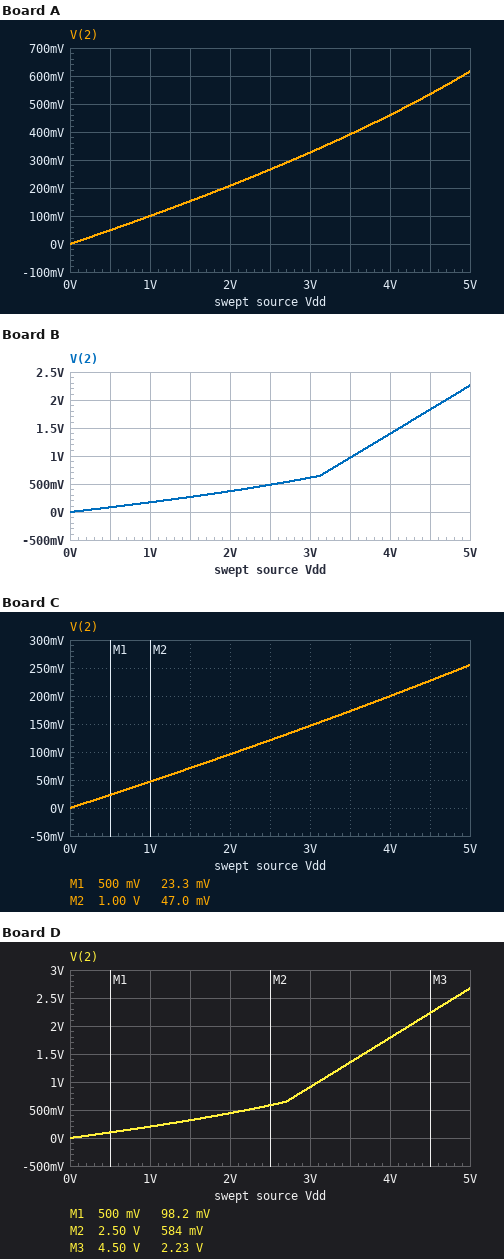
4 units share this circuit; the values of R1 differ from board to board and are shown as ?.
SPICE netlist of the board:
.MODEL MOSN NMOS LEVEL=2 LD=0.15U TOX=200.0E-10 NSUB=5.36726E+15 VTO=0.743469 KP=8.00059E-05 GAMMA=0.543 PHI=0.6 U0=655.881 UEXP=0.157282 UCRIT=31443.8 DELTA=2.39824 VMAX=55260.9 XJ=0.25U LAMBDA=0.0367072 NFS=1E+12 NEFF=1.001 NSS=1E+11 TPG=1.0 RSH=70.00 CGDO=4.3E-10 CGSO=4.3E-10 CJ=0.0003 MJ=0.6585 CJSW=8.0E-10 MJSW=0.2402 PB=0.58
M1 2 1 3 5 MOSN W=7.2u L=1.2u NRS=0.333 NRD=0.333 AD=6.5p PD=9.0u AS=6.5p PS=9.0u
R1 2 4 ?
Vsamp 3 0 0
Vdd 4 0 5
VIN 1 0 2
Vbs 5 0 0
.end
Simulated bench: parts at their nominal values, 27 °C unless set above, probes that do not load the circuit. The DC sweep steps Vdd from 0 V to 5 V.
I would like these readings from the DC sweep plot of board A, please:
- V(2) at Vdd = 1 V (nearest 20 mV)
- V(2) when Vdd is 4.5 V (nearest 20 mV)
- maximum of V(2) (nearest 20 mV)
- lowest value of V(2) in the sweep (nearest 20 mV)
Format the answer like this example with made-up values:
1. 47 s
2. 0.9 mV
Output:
1. 100 mV
2. 540 mV
3. 620 mV
4. 0 V
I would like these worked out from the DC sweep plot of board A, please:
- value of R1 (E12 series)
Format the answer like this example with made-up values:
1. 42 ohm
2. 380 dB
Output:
1. 15 kΩ
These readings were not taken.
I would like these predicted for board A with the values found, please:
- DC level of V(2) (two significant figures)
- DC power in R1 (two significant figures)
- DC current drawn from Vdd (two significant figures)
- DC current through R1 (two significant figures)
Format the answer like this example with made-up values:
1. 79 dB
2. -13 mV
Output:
1. 620 mV
2. 1.3 mW
3. 290 µA
4. 290 µA
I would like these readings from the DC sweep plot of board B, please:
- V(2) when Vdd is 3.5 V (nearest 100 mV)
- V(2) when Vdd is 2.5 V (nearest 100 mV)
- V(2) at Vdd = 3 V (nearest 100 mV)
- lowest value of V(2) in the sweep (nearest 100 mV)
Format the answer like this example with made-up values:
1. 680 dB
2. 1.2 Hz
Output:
1. 1.0 V
2. 500 mV
3. 600 mV
4. 0 V
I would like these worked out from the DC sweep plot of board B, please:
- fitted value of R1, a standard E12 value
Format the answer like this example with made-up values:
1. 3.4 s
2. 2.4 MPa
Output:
1. 8.2 kΩ
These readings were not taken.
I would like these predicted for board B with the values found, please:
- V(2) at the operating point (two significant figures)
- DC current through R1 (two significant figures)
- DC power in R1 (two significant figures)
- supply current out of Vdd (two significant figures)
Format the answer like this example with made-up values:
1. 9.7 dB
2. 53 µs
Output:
1. 2.3 V
2. 330 µA
3. 920 µW
4. 330 µA
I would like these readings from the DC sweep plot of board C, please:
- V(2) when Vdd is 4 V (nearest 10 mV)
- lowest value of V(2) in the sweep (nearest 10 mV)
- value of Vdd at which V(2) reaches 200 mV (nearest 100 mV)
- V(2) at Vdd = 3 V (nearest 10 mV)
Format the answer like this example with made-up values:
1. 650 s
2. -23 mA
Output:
1. 200 mV
2. 0 V
3. 4.0 V
4. 150 mV
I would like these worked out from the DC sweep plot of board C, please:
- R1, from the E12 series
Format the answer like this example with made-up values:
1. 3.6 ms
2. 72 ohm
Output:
1. 33 kΩ
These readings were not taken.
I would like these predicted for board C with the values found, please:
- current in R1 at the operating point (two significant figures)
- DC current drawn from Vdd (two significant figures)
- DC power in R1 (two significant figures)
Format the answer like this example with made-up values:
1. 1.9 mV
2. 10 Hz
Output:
1. 140 µA
2. 140 µA
3. 680 µW
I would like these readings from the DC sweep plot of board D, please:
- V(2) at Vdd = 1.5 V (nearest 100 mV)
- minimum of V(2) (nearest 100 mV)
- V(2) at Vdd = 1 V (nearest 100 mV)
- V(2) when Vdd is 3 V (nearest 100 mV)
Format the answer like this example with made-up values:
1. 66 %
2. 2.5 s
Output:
1. 300 mV
2. 0 V
3. 200 mV
4. 900 mV
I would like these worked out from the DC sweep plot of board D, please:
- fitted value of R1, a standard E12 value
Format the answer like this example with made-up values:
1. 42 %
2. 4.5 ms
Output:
1. 6.8 kΩ
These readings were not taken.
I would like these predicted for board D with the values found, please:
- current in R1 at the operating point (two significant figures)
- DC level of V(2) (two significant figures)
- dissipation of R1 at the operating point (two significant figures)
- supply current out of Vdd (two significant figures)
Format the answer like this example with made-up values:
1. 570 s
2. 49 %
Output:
1. 340 µA
2. 2.7 V
3. 800 µW
4. 340 µA
